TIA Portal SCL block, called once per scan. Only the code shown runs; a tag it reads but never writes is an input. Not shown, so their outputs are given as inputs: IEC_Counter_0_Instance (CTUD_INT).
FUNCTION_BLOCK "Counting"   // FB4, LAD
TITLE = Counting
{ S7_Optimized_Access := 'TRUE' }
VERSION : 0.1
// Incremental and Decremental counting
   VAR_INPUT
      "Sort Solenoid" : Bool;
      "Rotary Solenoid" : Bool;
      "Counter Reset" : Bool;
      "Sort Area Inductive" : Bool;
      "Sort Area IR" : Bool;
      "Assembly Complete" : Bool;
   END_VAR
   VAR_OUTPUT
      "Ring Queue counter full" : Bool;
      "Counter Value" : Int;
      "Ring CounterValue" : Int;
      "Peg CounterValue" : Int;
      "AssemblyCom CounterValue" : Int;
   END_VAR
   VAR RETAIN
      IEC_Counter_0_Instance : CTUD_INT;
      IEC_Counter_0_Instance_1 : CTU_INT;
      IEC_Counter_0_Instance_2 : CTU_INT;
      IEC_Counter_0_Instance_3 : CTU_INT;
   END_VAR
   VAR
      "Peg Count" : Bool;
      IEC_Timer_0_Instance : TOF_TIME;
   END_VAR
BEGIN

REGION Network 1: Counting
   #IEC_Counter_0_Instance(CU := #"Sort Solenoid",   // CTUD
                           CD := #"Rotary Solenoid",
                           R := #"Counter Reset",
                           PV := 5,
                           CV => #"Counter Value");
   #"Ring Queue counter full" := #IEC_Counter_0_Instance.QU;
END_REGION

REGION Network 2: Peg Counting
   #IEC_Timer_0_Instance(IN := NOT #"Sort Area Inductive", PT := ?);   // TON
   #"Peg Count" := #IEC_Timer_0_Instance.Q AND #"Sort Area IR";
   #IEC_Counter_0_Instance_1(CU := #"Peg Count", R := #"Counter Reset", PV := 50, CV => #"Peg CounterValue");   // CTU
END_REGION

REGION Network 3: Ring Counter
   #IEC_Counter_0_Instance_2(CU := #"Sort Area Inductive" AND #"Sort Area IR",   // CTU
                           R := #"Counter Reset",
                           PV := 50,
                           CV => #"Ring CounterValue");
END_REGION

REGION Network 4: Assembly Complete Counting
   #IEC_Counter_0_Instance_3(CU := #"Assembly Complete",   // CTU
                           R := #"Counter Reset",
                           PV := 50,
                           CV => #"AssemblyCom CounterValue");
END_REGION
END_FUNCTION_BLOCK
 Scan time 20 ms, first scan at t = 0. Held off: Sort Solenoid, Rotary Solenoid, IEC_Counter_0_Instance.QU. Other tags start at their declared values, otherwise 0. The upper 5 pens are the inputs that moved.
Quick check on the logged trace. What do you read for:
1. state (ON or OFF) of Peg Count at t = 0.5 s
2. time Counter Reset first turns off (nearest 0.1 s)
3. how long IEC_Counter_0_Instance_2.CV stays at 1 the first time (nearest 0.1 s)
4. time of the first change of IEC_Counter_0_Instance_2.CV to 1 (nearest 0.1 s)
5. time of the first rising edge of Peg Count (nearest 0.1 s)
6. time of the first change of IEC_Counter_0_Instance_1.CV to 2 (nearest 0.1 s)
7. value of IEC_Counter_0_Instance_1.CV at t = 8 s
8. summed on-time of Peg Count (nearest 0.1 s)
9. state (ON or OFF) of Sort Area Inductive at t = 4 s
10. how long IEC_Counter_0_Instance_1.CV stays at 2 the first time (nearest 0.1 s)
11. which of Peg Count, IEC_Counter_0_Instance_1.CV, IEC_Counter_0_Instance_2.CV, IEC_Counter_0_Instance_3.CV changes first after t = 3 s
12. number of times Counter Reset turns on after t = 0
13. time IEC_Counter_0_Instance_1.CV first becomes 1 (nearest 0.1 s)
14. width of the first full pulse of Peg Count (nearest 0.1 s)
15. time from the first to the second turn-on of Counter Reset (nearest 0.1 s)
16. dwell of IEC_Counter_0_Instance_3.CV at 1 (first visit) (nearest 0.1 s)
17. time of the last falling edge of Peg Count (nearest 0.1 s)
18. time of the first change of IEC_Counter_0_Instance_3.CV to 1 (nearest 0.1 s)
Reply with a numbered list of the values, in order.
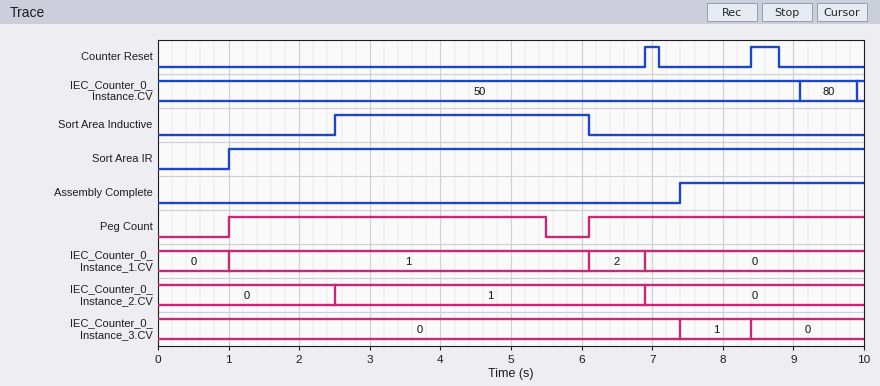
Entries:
1. OFF
2. 7.1 s
3. 4.4 s
4. 2.5 s
5. 1.0 s
6. 6.1 s
7. 0
8. 8.4 s
9. ON
10. 0.8 s
11. Peg Count
12. 2
13. 1.0 s
14. 4.5 s
15. 1.5 s
16. 1.0 s
17. 5.5 s
18. 7.4 s
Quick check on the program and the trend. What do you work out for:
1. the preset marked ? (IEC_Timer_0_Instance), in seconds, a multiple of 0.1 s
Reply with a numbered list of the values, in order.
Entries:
1. 3.0 s
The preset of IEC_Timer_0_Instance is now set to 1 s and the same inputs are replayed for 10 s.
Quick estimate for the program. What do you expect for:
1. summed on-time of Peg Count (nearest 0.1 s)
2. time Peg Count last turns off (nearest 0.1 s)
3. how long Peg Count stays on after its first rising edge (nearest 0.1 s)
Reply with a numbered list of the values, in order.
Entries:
1. 6.4 s
2. 3.5 s
3. 2.5 s
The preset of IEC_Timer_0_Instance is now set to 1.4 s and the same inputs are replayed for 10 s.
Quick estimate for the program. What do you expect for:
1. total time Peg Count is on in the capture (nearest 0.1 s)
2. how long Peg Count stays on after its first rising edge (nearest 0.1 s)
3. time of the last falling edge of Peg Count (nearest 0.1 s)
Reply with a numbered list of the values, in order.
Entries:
1. 6.8 s
2. 2.9 s
3. 3.9 s
